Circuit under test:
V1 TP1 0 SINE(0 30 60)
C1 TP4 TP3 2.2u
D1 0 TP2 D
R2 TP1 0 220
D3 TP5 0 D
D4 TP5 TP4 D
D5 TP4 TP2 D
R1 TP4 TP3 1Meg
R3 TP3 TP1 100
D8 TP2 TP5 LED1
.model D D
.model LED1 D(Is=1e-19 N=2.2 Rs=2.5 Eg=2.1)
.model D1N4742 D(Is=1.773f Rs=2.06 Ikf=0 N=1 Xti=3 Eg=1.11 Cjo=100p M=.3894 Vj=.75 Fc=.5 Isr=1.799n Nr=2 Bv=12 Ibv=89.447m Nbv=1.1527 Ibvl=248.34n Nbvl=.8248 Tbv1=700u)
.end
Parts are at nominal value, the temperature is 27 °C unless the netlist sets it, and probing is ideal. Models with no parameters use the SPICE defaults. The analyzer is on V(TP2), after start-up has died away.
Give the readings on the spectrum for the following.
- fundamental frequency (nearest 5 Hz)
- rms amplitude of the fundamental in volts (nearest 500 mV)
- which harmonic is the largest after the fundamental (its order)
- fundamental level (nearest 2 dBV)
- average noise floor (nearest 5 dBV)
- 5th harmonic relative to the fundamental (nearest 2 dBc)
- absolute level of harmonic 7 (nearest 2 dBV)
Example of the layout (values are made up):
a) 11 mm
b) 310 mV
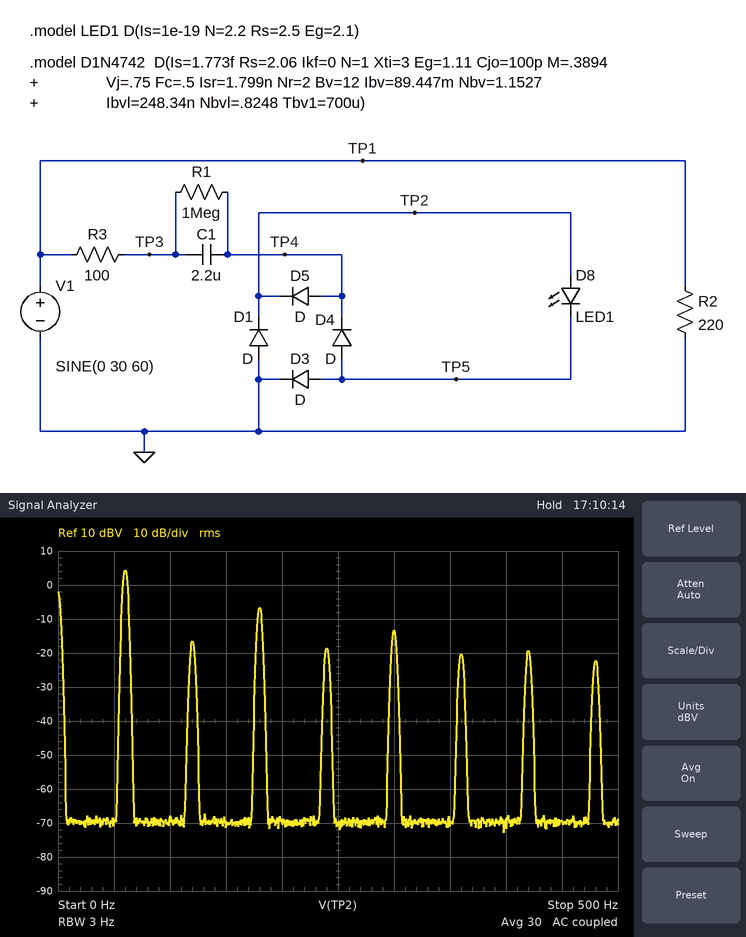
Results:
a) 60 Hz
b) 1.5 V
c) 3
d) 4 dBV
e) -70 dBV
f) -18 dBc
g) -20 dBV
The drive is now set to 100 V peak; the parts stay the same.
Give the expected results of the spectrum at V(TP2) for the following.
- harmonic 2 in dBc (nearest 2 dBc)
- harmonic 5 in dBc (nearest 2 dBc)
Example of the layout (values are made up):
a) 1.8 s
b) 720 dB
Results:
a) -24 dBc
b) -16 dBc
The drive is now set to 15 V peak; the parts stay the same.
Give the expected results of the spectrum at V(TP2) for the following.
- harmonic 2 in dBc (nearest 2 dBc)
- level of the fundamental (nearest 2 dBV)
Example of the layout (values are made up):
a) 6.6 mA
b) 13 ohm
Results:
a) -18 dBc
b) 4 dBV
